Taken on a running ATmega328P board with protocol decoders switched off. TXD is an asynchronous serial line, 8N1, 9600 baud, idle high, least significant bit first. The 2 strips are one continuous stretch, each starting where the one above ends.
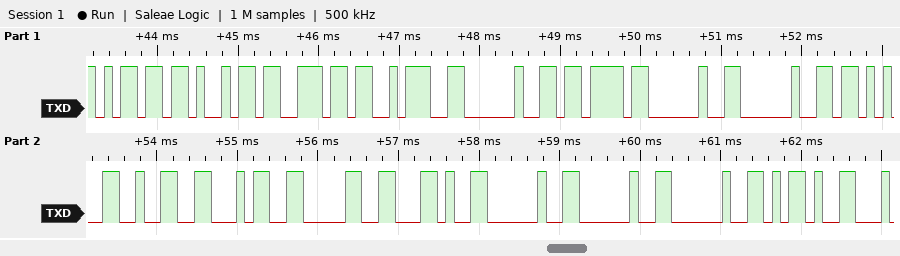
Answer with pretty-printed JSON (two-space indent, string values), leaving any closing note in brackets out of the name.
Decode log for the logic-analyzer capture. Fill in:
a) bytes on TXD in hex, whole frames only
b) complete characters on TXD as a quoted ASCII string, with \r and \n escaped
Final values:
{
  "bytes on TXD in hex, whole frames only": "6D 69 6E 3A 20 7B 20 20 2B 32 34 30 2C 20 20 20 2D",
  "complete characters on TXD as a quoted ASCII string, with \\r and \\n escaped": "\"min: {  +240,   -\""
}
